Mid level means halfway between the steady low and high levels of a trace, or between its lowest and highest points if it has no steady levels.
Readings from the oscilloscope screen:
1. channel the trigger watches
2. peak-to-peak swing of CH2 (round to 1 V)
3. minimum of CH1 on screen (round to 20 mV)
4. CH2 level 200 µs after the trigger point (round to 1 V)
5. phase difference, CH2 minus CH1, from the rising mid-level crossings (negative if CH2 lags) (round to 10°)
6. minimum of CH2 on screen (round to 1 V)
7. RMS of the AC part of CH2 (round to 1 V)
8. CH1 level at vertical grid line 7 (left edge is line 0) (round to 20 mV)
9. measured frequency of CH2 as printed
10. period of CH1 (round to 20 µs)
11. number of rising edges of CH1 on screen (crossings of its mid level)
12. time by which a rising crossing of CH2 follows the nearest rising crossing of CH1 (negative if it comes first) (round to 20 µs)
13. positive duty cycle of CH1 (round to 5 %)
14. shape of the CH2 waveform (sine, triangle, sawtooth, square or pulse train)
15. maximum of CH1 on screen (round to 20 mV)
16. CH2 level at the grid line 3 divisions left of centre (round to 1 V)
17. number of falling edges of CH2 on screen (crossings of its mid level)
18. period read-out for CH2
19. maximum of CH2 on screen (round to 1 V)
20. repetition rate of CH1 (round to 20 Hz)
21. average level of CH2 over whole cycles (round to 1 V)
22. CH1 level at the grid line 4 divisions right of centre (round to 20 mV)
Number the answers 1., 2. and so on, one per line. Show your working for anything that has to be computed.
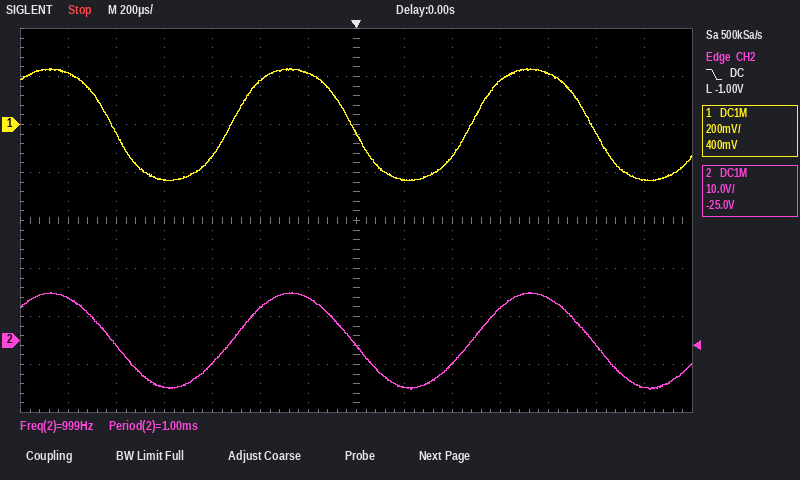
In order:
1. CH2
2. 10 V − (-10 V) = 20 V
3. -240 mV
4. -10 V
5. −360° × (0 µs) / 1.00 ms ≈ 0°
6. -10 V
7. 20 V / (2√2) ≈ 7 V
8. -40 mV
9. 999 Hz
10. 1.00 ms
11. 2
12. 0 µs
13. 50 %
14. sine
15. 240 mV
16. -5 V
17. 3
18. 1.00 ms
19. 10 V
20. 1 / 1.00 ms ≈ 1.00 kHz
21. (10 V + (-10 V)) / 2 ≈ 0 V
22. 220 mV
